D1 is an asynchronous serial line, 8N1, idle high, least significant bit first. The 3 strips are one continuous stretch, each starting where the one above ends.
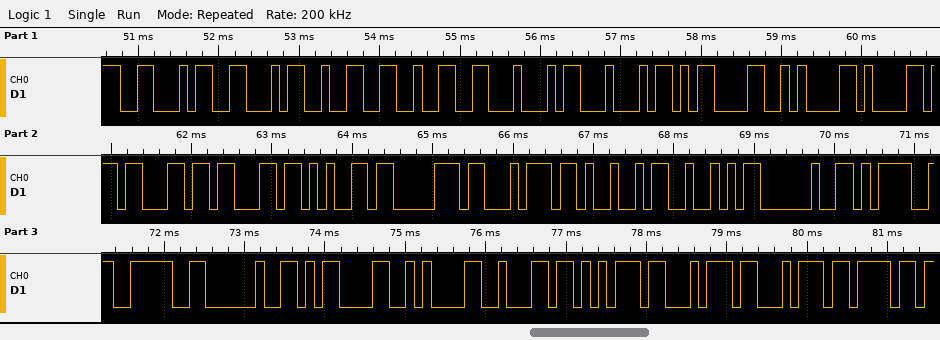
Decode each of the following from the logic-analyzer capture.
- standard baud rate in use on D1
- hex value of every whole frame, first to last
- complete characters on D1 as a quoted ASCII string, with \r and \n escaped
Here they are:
9600 baud
46 46 32 32 44 44 0D 0A 61 63 63 65 70 74 49 52 20 3D 3E 20 0D 0A 62 75 74 74 6F
"FF22DD\r\nacceptIR => \r\nbutto"
